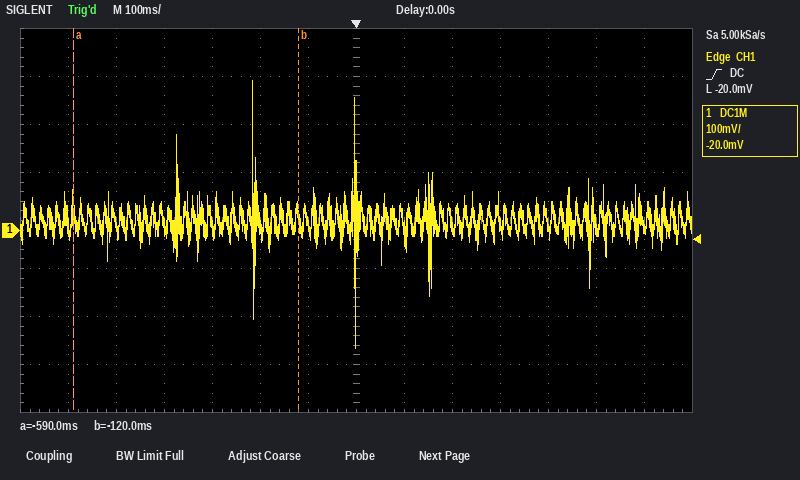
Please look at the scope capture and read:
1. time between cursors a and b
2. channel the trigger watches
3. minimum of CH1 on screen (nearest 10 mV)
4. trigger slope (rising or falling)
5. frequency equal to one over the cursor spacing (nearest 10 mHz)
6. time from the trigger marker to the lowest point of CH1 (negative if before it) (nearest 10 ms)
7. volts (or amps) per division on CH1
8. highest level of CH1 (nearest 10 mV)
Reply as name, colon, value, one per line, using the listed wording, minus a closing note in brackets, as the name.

time between cursors a and b: 470 ms
channel the trigger watches: CH1
minimum of CH1 on screen: -240 mV
trigger slope: rising
frequency equal to one over the cursor spacing: 2.13 Hz
time from the trigger marker to the lowest point of CH1 (negative if before it): 0 ms
volts (or amps) per division on CH1: 100 mV
highest level of CH1: 310 mV
